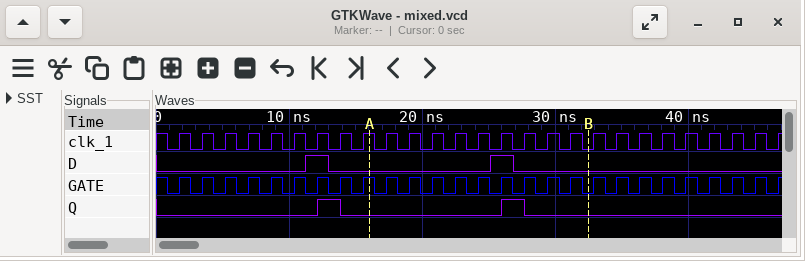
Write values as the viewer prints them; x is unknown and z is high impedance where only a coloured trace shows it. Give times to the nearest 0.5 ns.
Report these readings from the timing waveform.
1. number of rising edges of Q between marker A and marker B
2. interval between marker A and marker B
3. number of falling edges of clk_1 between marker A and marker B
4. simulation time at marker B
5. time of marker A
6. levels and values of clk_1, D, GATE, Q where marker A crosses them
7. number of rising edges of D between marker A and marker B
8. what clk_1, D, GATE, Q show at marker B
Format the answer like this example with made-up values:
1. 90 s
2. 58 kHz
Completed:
1. 1
2. 16.5 ns
3. 10
4. 32.5 ns
5. 16 ns
6. clk_1=1, D=0, GATE=1, Q=0
7. 1
8. clk_1=0, D=0, GATE=0, Q=0
